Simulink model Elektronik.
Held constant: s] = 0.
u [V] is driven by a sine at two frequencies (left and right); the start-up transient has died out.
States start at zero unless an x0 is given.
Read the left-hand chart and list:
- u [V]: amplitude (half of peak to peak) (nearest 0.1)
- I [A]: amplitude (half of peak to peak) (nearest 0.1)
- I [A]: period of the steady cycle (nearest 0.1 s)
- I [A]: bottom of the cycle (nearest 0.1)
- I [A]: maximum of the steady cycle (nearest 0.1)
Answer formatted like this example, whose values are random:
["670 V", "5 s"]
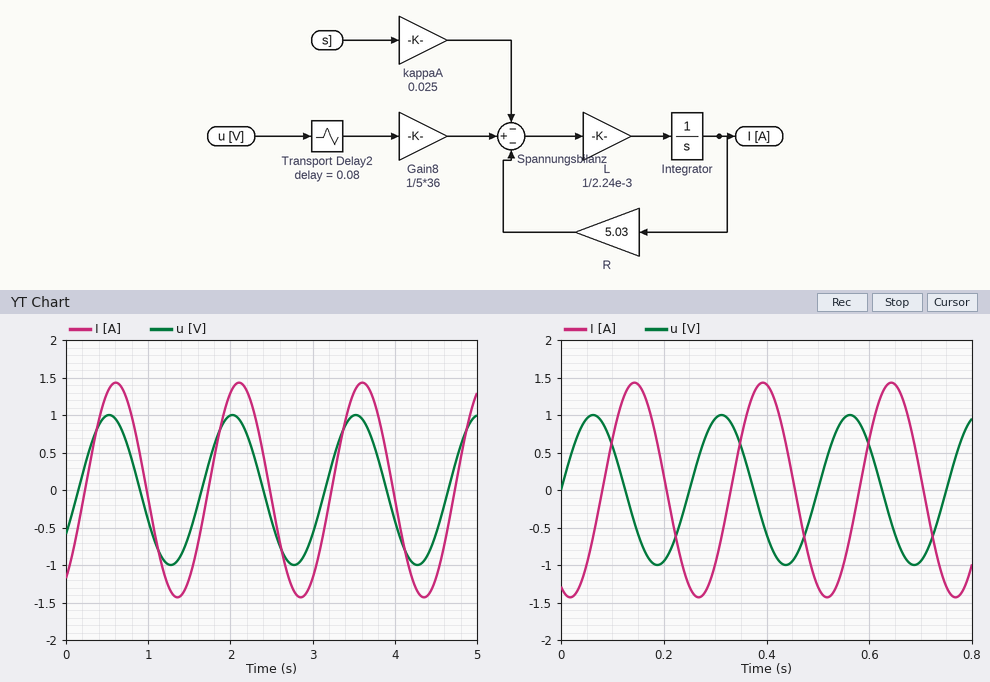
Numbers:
["1.0", "1.4", "1.5 s", "-1.4", "1.4"]
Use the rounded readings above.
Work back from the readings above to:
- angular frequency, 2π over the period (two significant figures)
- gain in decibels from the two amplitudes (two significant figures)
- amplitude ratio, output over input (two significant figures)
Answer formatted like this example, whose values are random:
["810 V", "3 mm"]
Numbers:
["4.2 rad/s", "2.9 dB", "1.4"]
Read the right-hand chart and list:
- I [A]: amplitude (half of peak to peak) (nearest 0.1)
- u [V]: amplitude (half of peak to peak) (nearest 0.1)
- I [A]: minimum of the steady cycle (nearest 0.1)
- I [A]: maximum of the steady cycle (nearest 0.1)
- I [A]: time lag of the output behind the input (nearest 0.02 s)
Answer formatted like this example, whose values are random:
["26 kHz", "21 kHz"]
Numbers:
["1.4", "1.0", "-1.4", "1.4", "0.08 s"]
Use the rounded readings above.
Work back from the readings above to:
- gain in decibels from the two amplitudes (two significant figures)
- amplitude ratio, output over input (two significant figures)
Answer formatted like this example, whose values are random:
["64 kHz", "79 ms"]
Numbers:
["2.9 dB", "1.4"]
